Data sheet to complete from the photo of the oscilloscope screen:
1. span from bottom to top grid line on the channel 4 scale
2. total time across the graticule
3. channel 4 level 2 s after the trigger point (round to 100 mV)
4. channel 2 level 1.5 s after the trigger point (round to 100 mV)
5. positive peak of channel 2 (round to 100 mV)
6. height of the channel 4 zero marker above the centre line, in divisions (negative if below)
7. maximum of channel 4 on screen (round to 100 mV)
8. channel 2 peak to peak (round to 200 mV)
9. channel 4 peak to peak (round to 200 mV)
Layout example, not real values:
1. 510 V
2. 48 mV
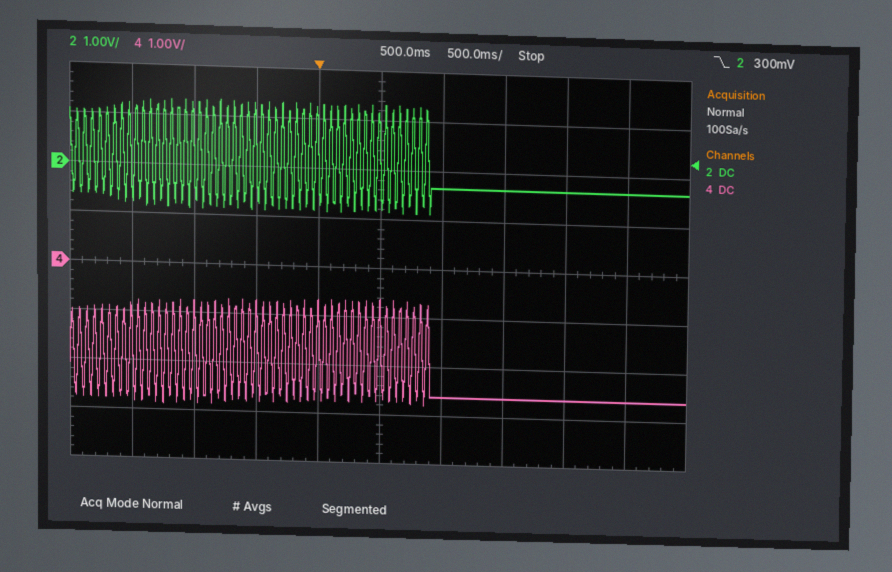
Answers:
1. 8 V
2. 5 s
3. -2.6 V
4. -300 mV
5. 1.3 V
6. 0.0 div
7. -600 mV
8. 2.2 V
9. 2.2 V
